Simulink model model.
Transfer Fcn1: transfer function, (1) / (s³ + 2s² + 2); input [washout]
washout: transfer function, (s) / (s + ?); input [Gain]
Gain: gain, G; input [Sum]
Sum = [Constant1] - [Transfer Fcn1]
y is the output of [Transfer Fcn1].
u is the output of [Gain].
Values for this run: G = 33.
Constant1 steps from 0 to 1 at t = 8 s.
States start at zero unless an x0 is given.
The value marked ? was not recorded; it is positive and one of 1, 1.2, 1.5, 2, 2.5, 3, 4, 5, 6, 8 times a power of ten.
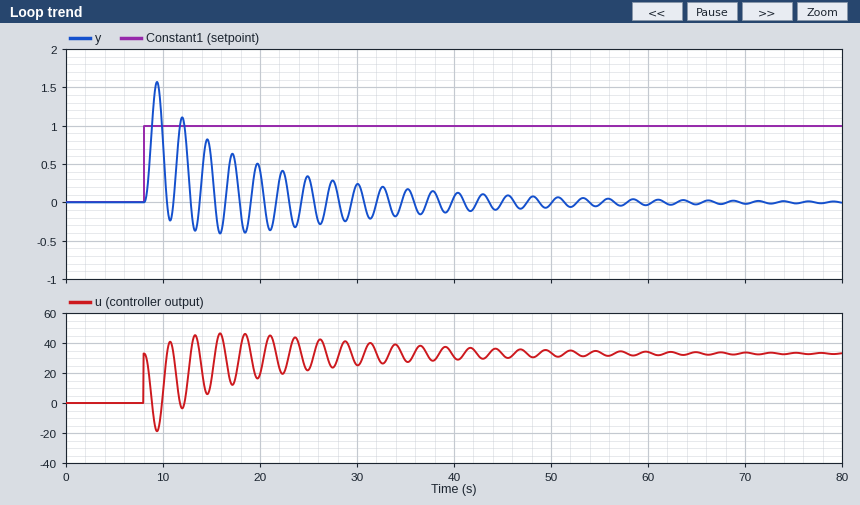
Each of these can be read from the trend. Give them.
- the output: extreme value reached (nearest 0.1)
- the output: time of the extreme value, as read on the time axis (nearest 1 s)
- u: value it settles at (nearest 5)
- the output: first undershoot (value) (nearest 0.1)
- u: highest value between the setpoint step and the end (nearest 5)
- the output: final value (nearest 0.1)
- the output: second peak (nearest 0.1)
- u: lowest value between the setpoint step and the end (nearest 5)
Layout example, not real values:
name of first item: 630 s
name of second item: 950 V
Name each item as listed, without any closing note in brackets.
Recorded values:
the output: extreme value reached: 1.6
the output: time of the extreme value, as read on the time axis: 9 s
u: value it settles at: 35
the output: first undershoot (value): -0.2
u: highest value between the setpoint step and the end: 45
the output: final value: 0.0
the output: second peak: 1.1
u: lowest value between the setpoint step and the end: -20
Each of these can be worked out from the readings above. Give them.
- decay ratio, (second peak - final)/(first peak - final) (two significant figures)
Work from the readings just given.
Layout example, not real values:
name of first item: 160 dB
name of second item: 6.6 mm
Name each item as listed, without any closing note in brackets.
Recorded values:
decay ratio, (second peak - final)/(first peak - final): 0.69
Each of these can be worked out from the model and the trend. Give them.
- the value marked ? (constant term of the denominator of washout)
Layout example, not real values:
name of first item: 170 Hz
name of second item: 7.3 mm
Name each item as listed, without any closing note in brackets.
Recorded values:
the value marked ?: 4
